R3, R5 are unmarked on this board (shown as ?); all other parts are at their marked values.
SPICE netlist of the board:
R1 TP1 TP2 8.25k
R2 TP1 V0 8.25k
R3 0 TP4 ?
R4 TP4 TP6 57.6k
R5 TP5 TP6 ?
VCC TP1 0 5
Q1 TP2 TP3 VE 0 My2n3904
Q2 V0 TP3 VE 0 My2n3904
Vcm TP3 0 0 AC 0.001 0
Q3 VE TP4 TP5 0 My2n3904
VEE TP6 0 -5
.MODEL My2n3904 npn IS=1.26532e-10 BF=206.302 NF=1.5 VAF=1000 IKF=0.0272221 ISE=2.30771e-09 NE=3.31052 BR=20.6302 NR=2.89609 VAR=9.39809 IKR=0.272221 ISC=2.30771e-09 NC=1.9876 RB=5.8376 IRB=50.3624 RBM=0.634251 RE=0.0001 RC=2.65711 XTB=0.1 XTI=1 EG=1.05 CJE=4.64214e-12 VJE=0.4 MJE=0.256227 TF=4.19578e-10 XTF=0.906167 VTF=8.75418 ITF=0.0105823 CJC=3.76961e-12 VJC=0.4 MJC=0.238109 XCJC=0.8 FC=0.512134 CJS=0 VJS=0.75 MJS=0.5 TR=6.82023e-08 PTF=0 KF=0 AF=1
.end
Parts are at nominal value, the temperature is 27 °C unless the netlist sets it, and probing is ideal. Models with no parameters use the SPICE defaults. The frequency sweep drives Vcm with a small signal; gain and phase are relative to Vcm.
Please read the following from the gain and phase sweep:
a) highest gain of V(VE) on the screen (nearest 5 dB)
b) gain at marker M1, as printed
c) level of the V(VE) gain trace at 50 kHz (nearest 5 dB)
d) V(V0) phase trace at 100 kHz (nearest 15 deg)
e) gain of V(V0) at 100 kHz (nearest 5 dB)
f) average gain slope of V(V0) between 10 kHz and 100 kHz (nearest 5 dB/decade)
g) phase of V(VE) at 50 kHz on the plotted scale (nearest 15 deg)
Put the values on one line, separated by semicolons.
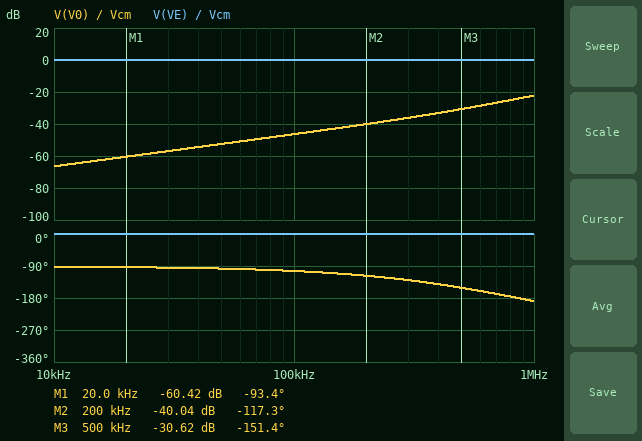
0 dB; -60.42 dB; 0 dB; -105 deg; -45 dB; 20 dB/decade; 0 deg
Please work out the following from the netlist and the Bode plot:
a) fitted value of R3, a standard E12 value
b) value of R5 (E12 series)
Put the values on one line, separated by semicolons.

120 kΩ; 22 kΩ
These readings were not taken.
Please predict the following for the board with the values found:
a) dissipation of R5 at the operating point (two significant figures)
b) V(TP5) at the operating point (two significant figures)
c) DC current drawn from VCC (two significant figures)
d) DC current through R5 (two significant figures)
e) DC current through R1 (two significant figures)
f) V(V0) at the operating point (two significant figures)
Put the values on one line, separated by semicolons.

53 µW; -3.9 V; 47 µA; 49 µA; 23 µA; 4.8 V
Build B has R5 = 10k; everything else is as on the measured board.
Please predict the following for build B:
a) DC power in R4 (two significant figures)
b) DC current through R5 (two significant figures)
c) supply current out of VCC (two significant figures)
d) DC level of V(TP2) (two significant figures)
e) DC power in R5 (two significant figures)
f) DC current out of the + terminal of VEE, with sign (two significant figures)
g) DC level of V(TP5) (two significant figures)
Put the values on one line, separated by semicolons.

42 µW; 100 µA; 99 µA; 4.6 V; 110 µW; -130 µA; -4.0 V
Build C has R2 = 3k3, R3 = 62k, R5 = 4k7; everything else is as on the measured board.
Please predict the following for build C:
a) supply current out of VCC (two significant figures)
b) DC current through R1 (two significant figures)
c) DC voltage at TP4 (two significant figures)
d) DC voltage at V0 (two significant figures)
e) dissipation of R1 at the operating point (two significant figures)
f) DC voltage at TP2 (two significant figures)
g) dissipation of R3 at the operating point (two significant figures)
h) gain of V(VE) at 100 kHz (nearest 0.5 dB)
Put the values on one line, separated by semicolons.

360 µA; 180 µA; -2.7 V; 4.4 V; 260 µW; 3.5 V; 120 µW; 0 dB
